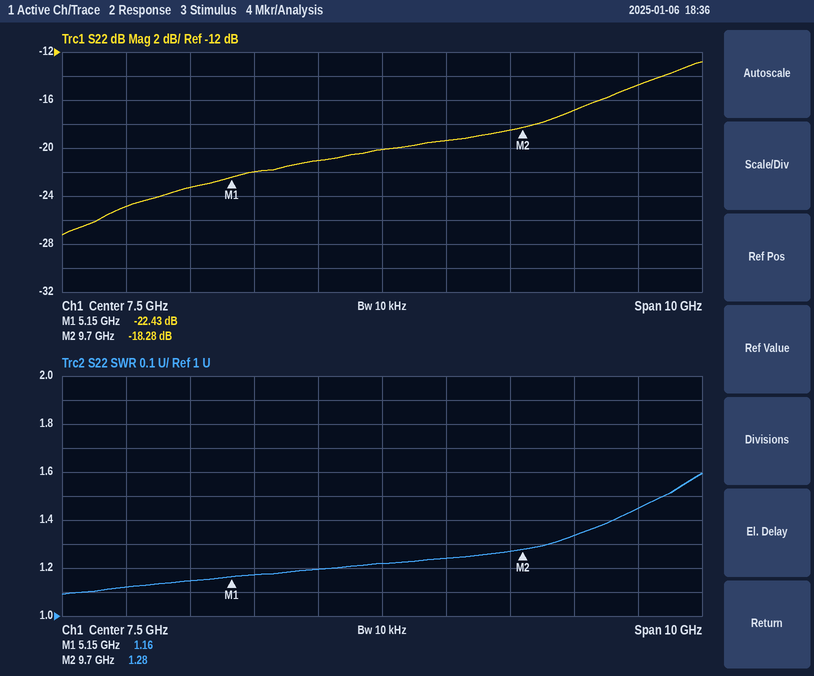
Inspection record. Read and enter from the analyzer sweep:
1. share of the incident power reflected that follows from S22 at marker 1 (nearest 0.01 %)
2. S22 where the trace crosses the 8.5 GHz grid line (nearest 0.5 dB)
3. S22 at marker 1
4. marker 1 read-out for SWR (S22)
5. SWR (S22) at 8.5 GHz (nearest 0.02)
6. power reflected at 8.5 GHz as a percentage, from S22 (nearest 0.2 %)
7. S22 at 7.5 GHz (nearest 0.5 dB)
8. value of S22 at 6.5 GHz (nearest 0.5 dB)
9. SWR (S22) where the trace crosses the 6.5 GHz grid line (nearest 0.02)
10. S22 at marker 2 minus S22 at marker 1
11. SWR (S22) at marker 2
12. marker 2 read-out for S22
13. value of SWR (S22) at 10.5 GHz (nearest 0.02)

0.57 %
-19.5 dB
-22.43 dB
1.16
1.24
1.2 %
-20.0 dB
-21.0 dB
1.20
4.15 dB
1.28
-18.28 dB
1.34
